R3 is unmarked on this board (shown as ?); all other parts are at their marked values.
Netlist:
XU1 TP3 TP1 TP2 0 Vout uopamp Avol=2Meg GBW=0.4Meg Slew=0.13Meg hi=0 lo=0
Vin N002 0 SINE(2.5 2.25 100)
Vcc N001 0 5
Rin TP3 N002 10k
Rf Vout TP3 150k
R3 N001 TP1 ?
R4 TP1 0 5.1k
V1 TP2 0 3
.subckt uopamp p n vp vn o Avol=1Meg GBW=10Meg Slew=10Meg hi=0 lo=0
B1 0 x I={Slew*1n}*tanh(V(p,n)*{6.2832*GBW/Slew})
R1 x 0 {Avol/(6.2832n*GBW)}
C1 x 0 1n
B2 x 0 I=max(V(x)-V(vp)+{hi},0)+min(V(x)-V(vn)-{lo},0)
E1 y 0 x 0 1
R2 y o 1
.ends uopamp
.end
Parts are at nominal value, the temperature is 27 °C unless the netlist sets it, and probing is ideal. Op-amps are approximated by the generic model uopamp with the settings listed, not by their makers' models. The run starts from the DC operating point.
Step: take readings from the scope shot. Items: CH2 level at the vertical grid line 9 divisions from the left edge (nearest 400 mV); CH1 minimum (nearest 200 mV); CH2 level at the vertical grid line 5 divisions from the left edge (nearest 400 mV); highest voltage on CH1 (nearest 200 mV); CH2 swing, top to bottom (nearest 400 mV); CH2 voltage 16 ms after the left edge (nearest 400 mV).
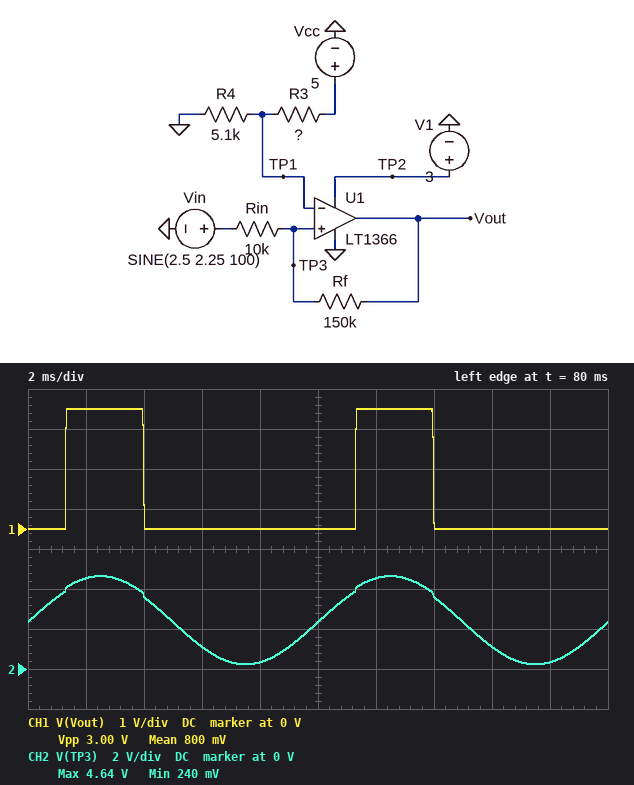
400 mV
0 V
2.4 V
3.0 V
4.4 V
1.2 V
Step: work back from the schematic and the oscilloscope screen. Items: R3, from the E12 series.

1.5 kΩ
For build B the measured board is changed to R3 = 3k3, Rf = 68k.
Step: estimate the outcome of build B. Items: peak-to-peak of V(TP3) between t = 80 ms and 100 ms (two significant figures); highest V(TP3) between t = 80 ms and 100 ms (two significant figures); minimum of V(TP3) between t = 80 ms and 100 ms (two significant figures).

4.3 V
4.5 V
220 mV
